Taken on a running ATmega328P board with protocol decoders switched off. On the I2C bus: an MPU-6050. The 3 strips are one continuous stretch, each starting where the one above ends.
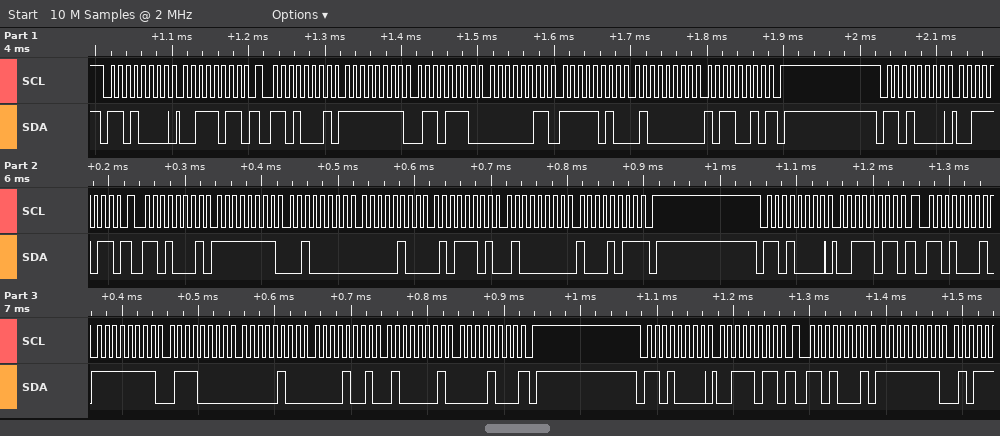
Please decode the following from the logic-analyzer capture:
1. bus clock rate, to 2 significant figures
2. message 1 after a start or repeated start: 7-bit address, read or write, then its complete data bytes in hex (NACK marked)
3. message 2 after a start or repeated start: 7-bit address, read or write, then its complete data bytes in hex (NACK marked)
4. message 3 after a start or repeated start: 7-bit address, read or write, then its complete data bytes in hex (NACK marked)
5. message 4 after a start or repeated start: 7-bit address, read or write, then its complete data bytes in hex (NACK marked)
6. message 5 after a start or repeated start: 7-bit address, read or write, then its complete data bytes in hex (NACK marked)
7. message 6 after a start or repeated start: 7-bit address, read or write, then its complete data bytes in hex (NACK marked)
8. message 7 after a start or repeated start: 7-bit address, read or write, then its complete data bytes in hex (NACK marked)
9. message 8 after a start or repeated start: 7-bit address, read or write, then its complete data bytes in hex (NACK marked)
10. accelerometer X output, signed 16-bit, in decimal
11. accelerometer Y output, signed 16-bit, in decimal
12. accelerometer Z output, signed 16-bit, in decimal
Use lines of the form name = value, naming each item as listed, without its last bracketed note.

bus clock rate, to 2 significant figures = 100 kHz
message 1 after a start or repeated start: 7-bit address, read or write, then its complete data bytes in hex = 0x68 write: 3B
message 2 after a start or repeated start: 7-bit address, read or write, then its complete data bytes in hex = 0x68 read: FF 6E 03 FA 40 B2 NACK
message 3 after a start or repeated start: 7-bit address, read or write, then its complete data bytes in hex = 0x68 write: 3B
message 4 after a start or repeated start: 7-bit address, read or write, then its complete data bytes in hex = 0x68 read: FF 20 04 5D 40 8B NACK
message 5 after a start or repeated start: 7-bit address, read or write, then its complete data bytes in hex = 0x68 write: 3B
message 6 after a start or repeated start: 7-bit address, read or write, then its complete data bytes in hex = 0x68 read: FF 70 04 09 41 08 NACK
message 7 after a start or repeated start: 7-bit address, read or write, then its complete data bytes in hex = 0x68 write: 3B
message 8 after a start or repeated start: 7-bit address, read or write, then its complete data bytes in hex = 0x68 read: FF
accelerometer X output, signed 16-bit, in decimal = -146
accelerometer Y output, signed 16-bit, in decimal = 1018
accelerometer Z output, signed 16-bit, in decimal = 16562
